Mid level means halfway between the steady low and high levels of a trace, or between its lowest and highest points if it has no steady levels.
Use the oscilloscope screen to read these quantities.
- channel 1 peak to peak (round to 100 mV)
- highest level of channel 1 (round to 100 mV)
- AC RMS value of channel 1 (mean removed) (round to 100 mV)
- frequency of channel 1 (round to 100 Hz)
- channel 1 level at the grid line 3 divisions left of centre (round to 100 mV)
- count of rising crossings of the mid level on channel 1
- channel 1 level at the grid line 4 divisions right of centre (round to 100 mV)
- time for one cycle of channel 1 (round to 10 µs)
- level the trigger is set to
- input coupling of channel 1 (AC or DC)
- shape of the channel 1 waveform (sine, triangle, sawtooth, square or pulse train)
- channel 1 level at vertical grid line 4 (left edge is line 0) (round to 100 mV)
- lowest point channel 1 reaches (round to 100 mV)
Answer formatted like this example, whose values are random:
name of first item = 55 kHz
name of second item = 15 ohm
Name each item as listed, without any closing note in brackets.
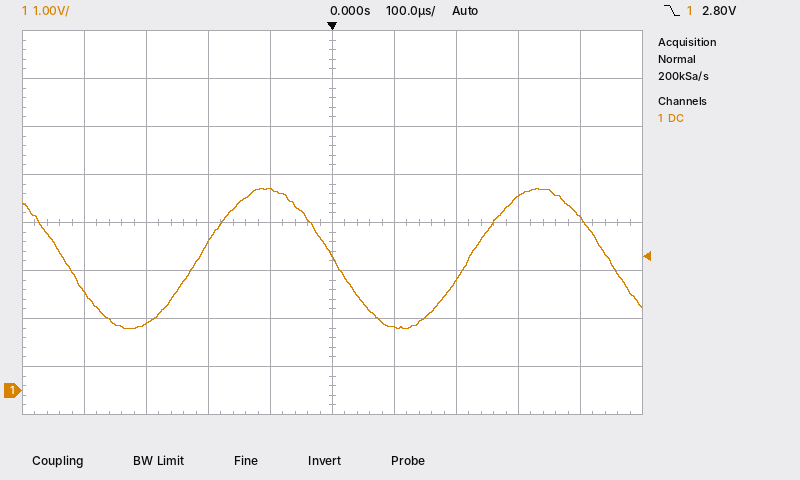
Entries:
channel 1 peak to peak = 2.9 V
highest level of channel 1 = 4.2 V
AC RMS value of channel 1 (mean removed) = 1.0 V
frequency of channel 1 = 2.3 kHz
channel 1 level at the grid line 3 divisions left of centre = 1.4 V
count of rising crossings of the mid level on channel 1 = 2
channel 1 level at the grid line 4 divisions right of centre = 3.6 V
time for one cycle of channel 1 = 440 µs
level the trigger is set to = 2.80 V
input coupling of channel 1 = DC
shape of the channel 1 waveform = sine
channel 1 level at vertical grid line 4 (left edge is line 0) = 4.2 V
lowest point channel 1 reaches = 1.3 V
